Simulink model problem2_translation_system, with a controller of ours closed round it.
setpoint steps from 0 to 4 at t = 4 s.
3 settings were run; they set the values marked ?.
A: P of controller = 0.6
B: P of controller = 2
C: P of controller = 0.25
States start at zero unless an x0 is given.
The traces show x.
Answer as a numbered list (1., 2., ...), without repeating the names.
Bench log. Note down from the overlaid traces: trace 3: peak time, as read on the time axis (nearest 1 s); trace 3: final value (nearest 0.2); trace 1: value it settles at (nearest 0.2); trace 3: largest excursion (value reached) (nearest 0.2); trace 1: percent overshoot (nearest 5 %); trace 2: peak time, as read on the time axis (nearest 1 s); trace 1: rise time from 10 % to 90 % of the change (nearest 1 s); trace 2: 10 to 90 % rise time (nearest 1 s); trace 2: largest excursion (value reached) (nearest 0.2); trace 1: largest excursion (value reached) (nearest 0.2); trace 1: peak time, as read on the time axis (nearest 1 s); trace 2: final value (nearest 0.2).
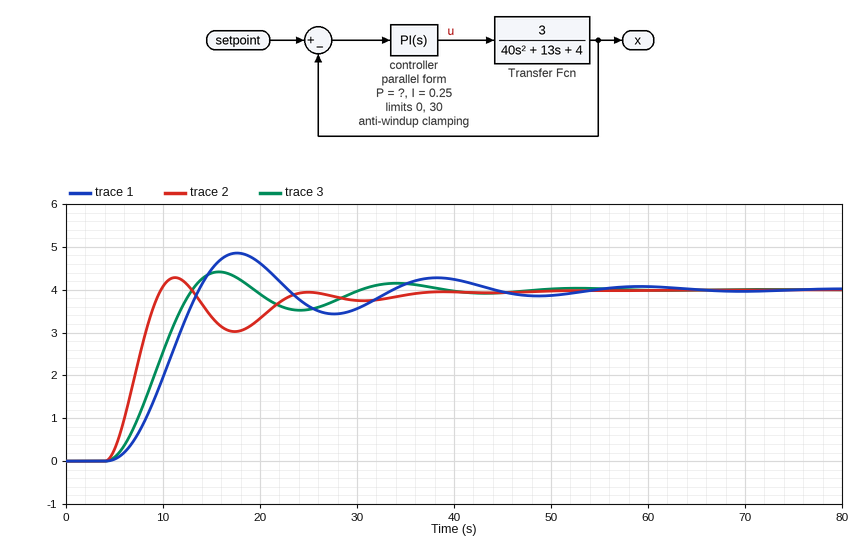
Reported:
1. 16 s
2. 4.0
3. 4.0
4. 4.4
5. 20 %
6. 11 s
7. 6 s
8. 4 s
9. 4.2
10. 4.8
11. 18 s
12. 4.0
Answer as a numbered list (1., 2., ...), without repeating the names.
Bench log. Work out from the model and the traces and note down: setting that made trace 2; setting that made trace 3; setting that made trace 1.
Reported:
1. B
2. A
3. C
